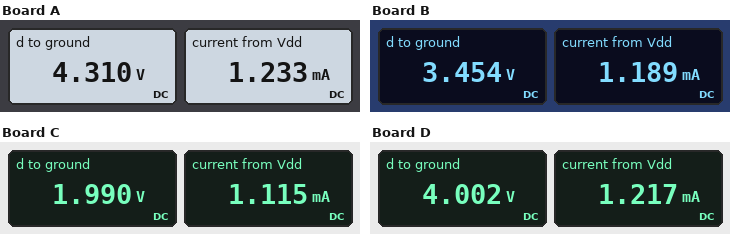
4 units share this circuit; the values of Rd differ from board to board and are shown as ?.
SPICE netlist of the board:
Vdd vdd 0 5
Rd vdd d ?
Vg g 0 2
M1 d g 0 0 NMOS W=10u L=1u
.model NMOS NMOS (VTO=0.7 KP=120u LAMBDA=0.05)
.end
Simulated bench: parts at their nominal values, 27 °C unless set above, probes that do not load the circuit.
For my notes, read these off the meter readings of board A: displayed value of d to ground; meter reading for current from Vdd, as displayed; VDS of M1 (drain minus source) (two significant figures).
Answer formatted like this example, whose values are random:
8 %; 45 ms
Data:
4.310 V; 1.233 mA; 4.3 V
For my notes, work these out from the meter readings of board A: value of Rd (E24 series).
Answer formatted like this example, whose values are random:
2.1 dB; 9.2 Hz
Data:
560 Ω
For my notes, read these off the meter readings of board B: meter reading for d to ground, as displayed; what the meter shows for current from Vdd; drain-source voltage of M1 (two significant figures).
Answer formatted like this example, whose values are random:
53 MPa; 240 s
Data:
3.454 V; 1.189 mA; 3.5 V
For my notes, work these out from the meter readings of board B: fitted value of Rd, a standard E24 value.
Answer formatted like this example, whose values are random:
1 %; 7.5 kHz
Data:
1.3 kΩ
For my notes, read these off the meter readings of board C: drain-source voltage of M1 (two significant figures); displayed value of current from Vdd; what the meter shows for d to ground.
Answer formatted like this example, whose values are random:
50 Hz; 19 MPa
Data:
2.0 V; 1.115 mA; 1.990 V
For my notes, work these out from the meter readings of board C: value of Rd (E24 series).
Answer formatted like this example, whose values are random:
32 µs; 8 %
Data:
2.7 kΩ
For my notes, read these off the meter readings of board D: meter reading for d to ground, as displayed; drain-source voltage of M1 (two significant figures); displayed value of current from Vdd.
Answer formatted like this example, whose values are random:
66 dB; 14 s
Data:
4.002 V; 4.0 V; 1.217 mA
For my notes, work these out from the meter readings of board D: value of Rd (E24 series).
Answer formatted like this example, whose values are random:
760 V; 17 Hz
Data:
820 Ω
